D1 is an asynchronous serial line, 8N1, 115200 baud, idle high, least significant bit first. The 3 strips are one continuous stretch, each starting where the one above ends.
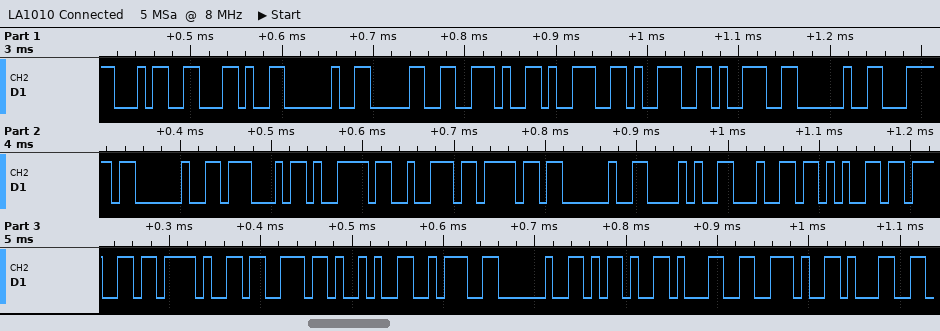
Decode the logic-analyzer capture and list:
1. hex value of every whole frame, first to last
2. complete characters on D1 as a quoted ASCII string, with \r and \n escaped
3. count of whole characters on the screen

34 2C 20 30 2E 39 39 39 20 7C 20 47 79 72 6F 20 28 64 65 67 2F 73 29 3A 20 2D 31 2E 31
"4, 0.999 | Gyro (deg/s): -1.1"
29
